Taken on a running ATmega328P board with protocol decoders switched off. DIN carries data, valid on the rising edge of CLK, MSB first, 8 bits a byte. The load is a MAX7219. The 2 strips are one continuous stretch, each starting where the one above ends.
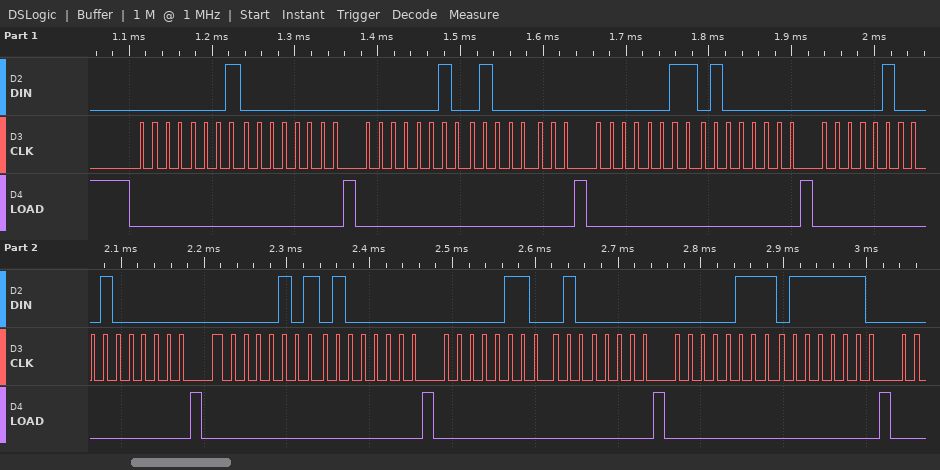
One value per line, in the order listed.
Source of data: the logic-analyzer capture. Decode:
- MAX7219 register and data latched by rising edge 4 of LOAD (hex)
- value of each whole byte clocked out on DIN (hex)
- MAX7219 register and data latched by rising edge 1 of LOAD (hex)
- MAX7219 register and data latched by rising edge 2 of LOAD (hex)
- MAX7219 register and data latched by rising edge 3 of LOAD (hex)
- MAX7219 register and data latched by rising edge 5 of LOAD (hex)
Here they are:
register 0x4, data 0x40
01 00 02 40 03 40 04 40 05 40 06 40 07 7E
register 0x1, data 0x00
register 0x2, data 0x40
register 0x3, data 0x40
register 0x5, data 0x40
